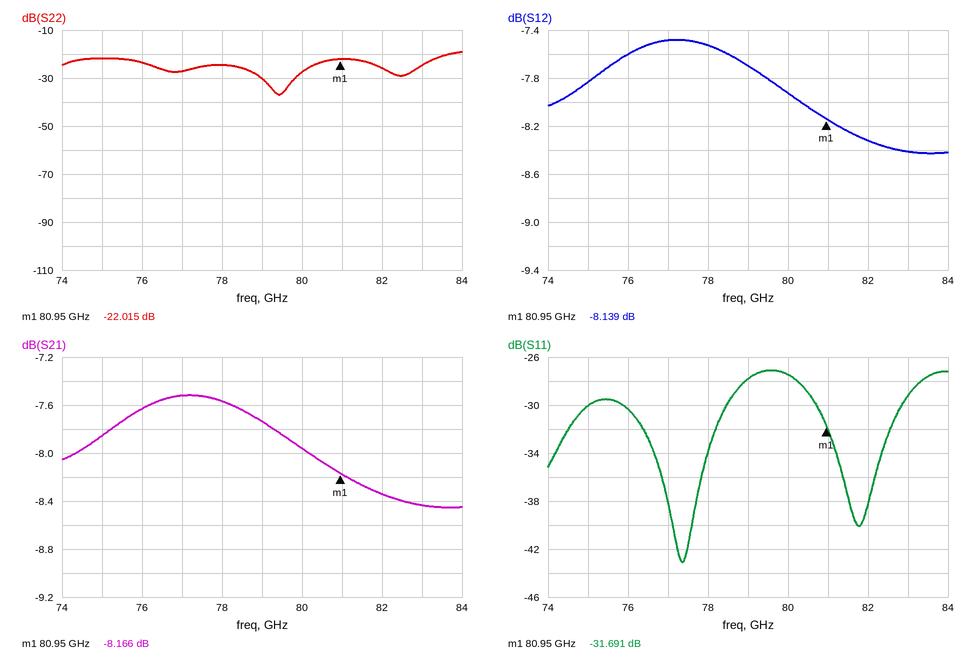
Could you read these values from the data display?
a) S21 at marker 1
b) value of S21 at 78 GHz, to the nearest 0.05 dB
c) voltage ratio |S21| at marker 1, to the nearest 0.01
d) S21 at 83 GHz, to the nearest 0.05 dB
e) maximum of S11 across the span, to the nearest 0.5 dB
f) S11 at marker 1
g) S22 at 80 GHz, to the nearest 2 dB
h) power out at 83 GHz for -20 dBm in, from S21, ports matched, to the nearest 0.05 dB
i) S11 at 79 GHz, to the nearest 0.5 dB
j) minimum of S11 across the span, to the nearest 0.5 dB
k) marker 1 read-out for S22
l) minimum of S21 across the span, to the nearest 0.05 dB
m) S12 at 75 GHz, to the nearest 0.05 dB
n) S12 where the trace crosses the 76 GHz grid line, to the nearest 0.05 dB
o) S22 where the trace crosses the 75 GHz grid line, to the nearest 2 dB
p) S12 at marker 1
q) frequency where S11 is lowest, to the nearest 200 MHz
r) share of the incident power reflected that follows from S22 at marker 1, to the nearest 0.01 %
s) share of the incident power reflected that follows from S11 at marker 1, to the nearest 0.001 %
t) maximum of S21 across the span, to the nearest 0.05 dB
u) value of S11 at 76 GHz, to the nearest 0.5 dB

-8.166 dB
-7.55 dB
0.39
-8.45 dB
-27.0 dB
-31.691 dB
-28 dB
-28.45 dBm
-28.0 dB
-43.0 dB
-22.015 dB
-8.45 dB
-7.85 dB
-7.60 dB
-22 dB
-8.139 dB
77.4 GHz
0.63 %
0.068 %
-7.50 dB
-30.5 dB
